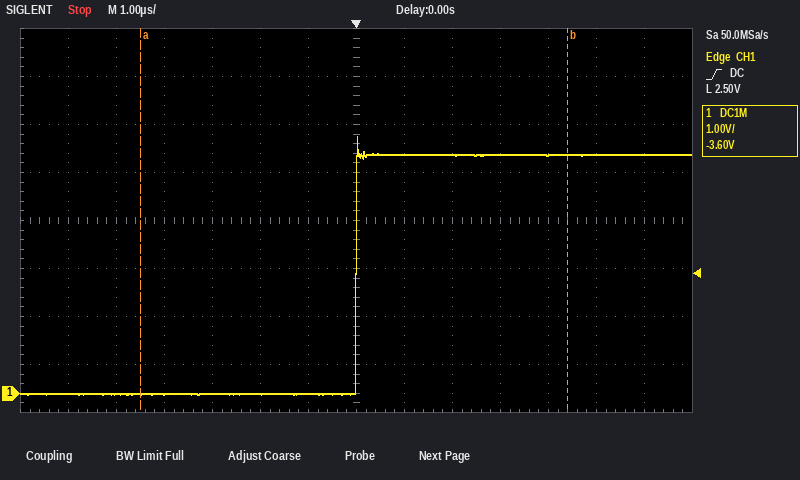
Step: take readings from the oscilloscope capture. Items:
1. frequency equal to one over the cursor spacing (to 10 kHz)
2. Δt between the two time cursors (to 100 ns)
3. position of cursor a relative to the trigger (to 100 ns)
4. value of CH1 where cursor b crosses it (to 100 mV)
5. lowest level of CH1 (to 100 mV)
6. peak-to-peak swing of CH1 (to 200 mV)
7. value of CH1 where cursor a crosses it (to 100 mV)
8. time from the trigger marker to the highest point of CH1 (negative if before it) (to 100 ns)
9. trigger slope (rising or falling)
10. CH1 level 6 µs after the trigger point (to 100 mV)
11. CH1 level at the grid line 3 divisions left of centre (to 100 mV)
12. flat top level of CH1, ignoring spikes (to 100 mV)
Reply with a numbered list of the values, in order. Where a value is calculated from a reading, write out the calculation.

1. 1 / 8.9 µs ≈ 110 kHz
2. 8.9 µs
3. -4.5 µs
4. 5.0 V
5. 0.0 V
6. 5.4 V
7. 0.0 V
8. 0.0 µs
9. rising
10. 5.0 V
11. 0.0 V
12. 5.0 V
